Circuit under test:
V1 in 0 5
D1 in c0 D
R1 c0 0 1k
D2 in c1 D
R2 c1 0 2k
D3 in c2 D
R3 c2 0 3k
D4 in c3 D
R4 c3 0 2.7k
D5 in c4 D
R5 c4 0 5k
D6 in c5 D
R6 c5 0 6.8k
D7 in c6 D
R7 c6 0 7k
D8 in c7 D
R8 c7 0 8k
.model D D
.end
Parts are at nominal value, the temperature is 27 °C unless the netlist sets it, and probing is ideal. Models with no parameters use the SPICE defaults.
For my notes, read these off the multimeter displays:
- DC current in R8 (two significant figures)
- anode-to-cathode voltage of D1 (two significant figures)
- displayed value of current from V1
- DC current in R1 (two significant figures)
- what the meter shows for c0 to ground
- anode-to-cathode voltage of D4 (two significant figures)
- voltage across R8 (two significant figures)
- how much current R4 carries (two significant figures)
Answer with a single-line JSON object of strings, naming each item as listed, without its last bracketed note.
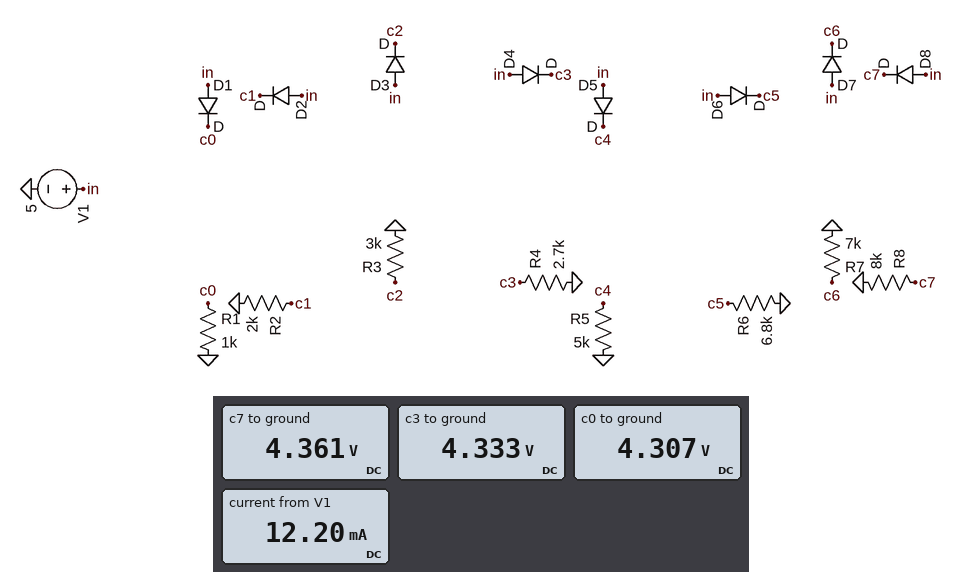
{"DC current in R8": "550 µA", "anode-to-cathode voltage of D1": "690 mV", "displayed value of current from V1": "12.20 mA", "DC current in R1": "4.3 mA", "what the meter shows for c0 to ground": "4.307 V", "anode-to-cathode voltage of D4": "670 mV", "voltage across R8": "4.4 V", "how much current R4 carries": "1.6 mA"}
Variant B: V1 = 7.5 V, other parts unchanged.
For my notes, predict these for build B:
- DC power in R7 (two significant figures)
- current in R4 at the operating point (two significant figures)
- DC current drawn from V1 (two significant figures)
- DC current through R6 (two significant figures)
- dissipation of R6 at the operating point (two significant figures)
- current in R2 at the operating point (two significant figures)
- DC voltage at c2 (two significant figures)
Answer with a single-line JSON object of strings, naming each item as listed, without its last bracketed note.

{"DC power in R7": "6.7 mW", "current in R4 at the operating point": "2.5 mA", "DC current drawn from V1": "19 mA", "DC current through R6": "1.0 mA", "dissipation of R6 at the operating point": "6.9 mW", "current in R2 at the operating point": "3.4 mA", "DC voltage at c2": "6.8 V"}
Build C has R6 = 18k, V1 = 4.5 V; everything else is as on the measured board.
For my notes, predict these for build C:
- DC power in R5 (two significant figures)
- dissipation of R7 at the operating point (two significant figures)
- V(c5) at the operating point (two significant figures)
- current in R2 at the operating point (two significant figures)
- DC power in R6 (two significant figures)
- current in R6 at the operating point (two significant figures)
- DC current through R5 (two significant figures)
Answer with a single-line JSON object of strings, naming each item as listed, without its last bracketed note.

{"DC power in R5": "3.0 mW", "dissipation of R7 at the operating point": "2.1 mW", "V(c5) at the operating point": "3.9 V", "current in R2 at the operating point": "1.9 mA", "DC power in R6": "840 µW", "current in R6 at the operating point": "220 µA", "DC current through R5": "770 µA"}
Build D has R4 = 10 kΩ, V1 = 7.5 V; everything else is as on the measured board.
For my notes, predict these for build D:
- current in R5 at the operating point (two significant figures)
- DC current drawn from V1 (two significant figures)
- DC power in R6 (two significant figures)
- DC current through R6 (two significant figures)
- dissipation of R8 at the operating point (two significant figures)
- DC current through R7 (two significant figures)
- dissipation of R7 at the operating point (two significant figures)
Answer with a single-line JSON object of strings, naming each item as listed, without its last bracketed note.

{"current in R5 at the operating point": "1.4 mA", "DC current drawn from V1": "17 mA", "DC power in R6": "6.9 mW", "DC current through R6": "1.0 mA", "dissipation of R8 at the operating point": "5.9 mW", "DC current through R7": "980 µA", "dissipation of R7 at the operating point": "6.7 mW"}
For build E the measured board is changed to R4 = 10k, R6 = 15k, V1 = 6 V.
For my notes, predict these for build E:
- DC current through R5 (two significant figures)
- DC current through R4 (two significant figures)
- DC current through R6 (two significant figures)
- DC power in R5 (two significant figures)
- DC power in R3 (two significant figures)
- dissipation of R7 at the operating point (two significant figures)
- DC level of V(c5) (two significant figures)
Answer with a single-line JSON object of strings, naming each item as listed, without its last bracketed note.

{"DC current through R5": "1.1 mA", "DC current through R4": "540 µA", "DC current through R6": "360 µA", "DC power in R5": "5.7 mW", "DC power in R3": "9.5 mW", "dissipation of R7 at the operating point": "4.1 mW", "DC level of V(c5)": "5.4 V"}
